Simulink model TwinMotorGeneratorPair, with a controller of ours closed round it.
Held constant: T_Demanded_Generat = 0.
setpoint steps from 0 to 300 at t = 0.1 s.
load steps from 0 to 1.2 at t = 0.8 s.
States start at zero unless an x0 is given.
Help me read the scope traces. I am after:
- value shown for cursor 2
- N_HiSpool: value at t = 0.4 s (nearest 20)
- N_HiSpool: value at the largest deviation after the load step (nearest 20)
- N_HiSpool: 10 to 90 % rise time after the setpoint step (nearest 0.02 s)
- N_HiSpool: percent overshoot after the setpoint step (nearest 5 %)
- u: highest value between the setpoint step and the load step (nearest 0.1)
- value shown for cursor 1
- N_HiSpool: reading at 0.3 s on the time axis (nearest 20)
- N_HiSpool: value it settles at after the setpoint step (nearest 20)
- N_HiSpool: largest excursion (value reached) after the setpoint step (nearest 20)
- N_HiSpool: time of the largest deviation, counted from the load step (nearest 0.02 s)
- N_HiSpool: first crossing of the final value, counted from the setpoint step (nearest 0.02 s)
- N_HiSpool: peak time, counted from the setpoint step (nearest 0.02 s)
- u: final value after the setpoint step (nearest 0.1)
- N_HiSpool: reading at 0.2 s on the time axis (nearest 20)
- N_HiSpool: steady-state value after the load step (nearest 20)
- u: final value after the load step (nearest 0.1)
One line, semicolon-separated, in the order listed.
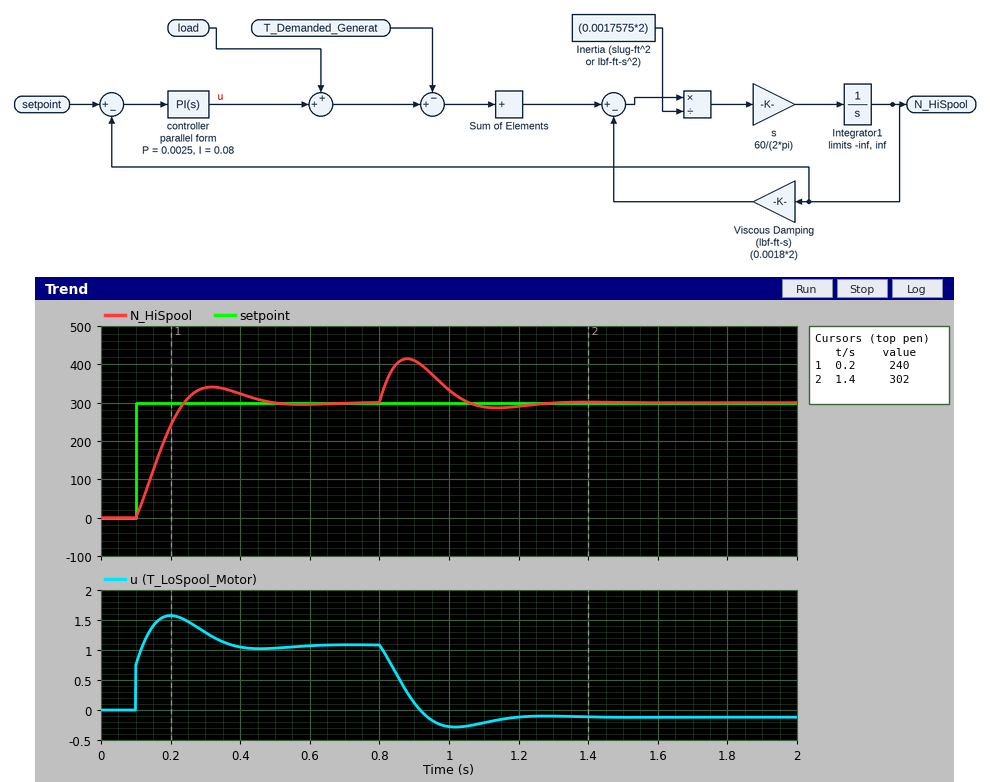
302; 320; 420; 0.10 s; 15 %; 1.6; 240; 340; 300; 340; 0.08 s; 0.14 s; 0.22 s; 1.1; 240; 300; -0.1
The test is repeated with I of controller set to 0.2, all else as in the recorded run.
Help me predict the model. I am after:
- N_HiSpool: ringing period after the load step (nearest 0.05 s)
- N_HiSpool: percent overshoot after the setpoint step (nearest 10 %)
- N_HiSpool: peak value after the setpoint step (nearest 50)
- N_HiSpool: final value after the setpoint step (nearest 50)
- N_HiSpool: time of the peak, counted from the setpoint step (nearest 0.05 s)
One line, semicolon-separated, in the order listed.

0.30 s; 30 %; 400; 300; 0.15 s
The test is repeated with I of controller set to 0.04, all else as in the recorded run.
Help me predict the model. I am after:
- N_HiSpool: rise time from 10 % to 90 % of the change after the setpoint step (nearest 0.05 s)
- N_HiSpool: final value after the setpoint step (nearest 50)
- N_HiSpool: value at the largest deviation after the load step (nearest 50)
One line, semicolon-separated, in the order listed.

0.20 s; 300; 450
